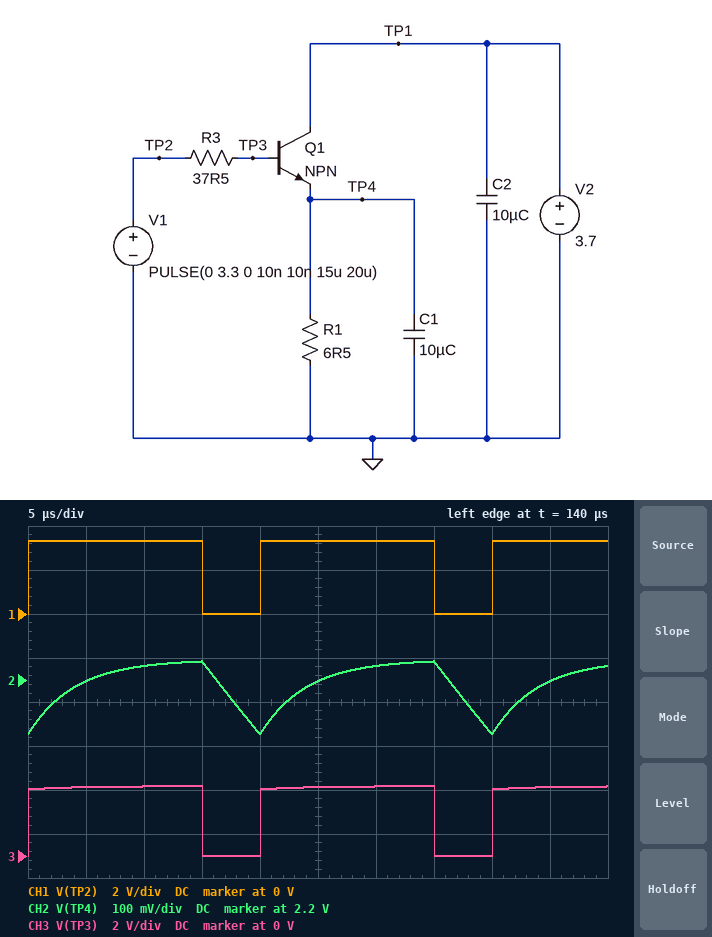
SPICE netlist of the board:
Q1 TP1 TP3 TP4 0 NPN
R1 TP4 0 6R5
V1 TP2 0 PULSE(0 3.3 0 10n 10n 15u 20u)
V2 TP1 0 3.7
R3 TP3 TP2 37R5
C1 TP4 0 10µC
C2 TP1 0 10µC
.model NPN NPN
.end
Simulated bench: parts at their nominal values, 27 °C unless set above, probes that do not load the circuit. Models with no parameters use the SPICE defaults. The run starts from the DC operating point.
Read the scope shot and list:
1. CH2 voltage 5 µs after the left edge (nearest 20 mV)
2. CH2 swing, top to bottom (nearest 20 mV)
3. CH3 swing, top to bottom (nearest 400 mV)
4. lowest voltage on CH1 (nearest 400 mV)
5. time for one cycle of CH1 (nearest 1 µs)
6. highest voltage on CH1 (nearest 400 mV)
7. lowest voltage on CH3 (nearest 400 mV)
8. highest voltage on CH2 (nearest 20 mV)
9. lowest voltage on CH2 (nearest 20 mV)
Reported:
2.20 V
160 mV
3.2 V
0 V
20 µs
3.2 V
0 V
2.24 V
2.08 V
